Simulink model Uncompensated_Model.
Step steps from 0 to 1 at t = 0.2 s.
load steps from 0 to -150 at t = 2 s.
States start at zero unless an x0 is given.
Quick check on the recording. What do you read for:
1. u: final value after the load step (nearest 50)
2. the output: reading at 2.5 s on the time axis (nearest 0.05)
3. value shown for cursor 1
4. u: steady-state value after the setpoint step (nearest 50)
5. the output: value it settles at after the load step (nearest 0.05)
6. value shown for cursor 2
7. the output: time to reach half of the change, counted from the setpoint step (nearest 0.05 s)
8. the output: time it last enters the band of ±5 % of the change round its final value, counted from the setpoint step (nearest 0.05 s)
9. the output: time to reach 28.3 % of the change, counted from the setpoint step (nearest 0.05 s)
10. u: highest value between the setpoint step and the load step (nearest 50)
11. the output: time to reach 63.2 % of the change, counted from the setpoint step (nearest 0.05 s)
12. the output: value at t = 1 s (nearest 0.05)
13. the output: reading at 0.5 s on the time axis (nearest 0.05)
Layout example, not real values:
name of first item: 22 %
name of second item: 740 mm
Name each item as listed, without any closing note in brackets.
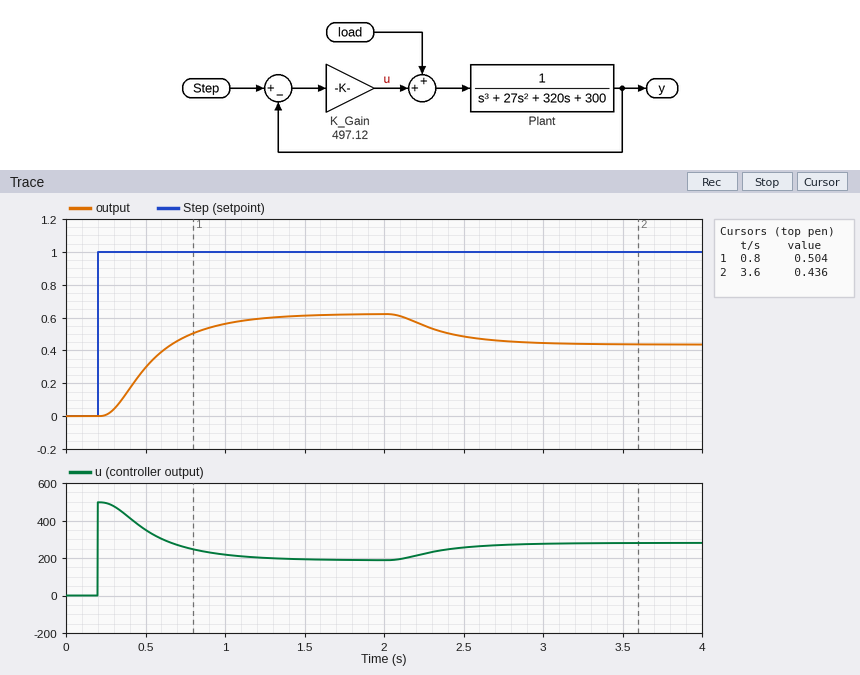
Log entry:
u: final value after the load step: 300
the output: reading at 2.5 s on the time axis: 0.50
value shown for cursor 1: 0.504
u: steady-state value after the setpoint step: 200
the output: value it settles at after the load step: 0.45
value shown for cursor 2: 0.436
the output: time to reach half of the change, counted from the setpoint step: 0.30 s
the output: time it last enters the band of ±5 % of the change round its final value, counted from the setpoint step: 1.00 s
the output: time to reach 28.3 % of the change, counted from the setpoint step: 0.20 s
u: highest value between the setpoint step and the load step: 500
the output: time to reach 63.2 % of the change, counted from the setpoint step: 0.40 s
the output: value at t = 1 s: 0.55
the output: reading at 0.5 s on the time axis: 0.30
